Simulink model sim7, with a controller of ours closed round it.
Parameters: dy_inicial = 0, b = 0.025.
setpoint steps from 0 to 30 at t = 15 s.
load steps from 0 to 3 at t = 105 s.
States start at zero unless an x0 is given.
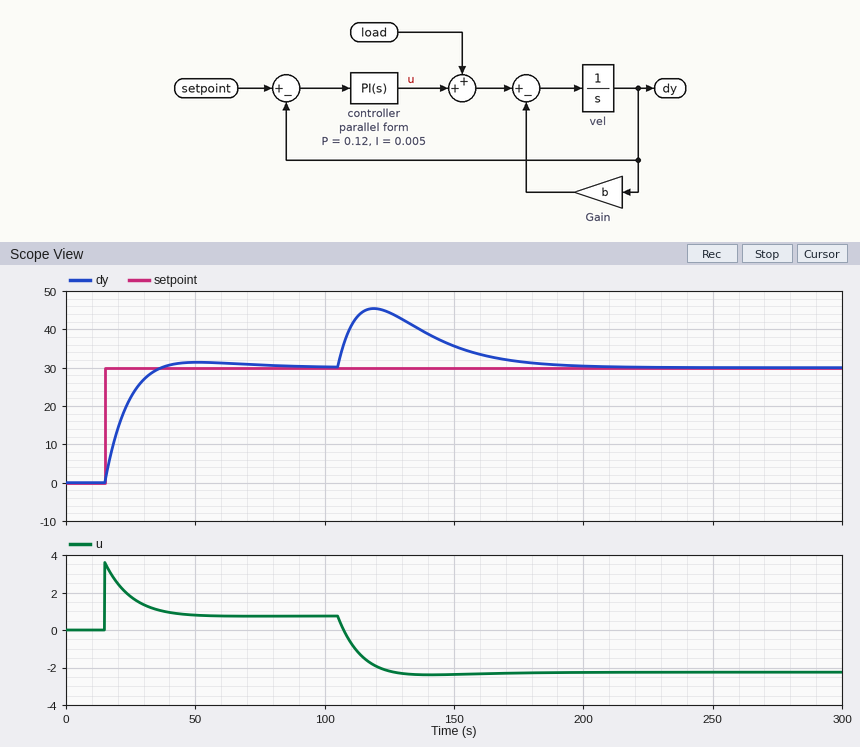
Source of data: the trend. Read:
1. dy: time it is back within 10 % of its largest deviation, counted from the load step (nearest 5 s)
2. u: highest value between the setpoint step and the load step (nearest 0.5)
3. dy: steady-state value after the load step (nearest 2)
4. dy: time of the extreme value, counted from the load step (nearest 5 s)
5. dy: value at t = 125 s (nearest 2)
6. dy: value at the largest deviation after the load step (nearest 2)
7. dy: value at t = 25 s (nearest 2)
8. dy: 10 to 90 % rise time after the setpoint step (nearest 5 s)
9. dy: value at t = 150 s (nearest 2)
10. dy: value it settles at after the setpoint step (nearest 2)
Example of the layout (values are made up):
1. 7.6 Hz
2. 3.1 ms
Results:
1. 70 s
2. 3.5
3. 30
4. 15 s
5. 44
6. 46
7. 22
8. 15 s
9. 36
10. 30
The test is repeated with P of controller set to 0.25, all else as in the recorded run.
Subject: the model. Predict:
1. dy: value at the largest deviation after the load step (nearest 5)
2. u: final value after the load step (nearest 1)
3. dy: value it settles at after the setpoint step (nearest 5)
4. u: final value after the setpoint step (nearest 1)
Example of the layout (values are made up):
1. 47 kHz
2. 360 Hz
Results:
1. 40
2. -2
3. 30
4. 1
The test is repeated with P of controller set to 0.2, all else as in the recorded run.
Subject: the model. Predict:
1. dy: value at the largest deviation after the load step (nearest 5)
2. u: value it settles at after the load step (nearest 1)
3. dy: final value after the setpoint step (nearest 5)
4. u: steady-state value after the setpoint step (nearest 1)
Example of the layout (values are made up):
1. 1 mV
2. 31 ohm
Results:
1. 40
2. -2
3. 30
4. 1
